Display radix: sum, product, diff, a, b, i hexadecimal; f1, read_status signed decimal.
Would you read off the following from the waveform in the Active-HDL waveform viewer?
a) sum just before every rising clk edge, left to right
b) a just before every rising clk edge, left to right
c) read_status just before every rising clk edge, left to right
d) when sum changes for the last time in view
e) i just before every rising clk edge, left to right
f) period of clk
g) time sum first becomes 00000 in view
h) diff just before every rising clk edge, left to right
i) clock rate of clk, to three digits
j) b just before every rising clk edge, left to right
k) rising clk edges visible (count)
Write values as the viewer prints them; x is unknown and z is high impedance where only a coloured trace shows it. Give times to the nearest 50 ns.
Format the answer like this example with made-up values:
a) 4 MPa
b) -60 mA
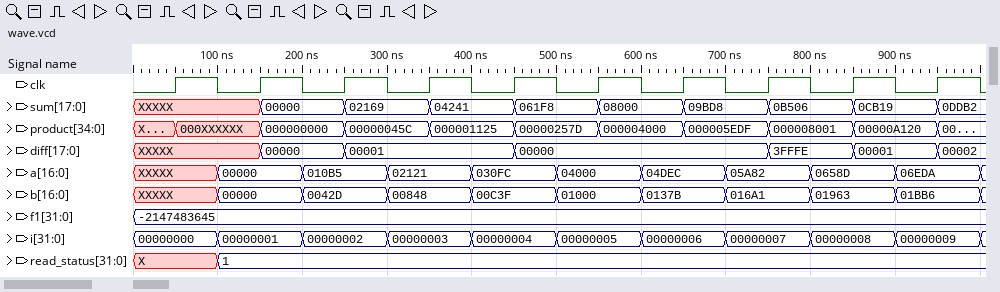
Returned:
a) XXXXX, XXXXX, 00000, 02169, 04241, 061F8, 08000, 09BD8, 0B506, 0CB19
b) XXXXX, 00000, 010B5, 02121, 030FC, 04000, 04DEC, 05A82, 0658D, 06EDA
c) X, 1, 1, 1, 1, 1, 1, 1, 1, 1
d) 950 ns
e) 00000000, 00000001, 00000002, 00000003, 00000004, 00000005, 00000006, 00000007, 00000008, 00000009
f) 100 ns
g) 150 ns
h) XXXXX, XXXXX, 00000, 00001, 00001, 00000, 00000, 00000, 3FFFE, 00001
i) 10.0 MHz
j) XXXXX, 00000, 0042D, 00848, 00C3F, 01000, 0137B, 016A1, 01963, 01BB6
k) 10
